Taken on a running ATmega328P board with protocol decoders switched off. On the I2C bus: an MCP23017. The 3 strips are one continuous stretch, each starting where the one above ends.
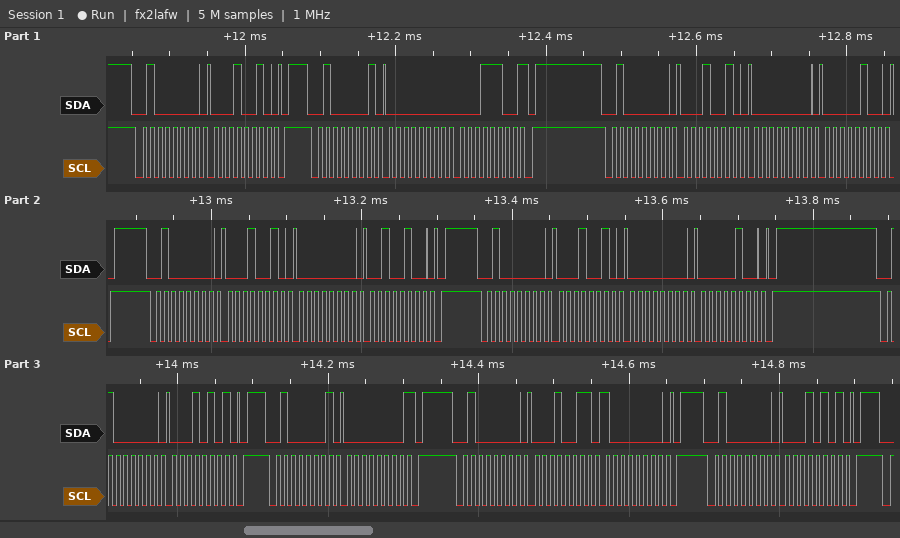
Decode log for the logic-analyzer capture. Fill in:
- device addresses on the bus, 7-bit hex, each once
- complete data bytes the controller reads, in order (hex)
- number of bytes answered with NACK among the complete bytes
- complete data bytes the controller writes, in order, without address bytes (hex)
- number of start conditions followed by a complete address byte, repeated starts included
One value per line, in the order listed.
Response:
0x20
00 1C 00
2
12 12 00 04 12 00 24 12 00 04 15 13 80 15
9
